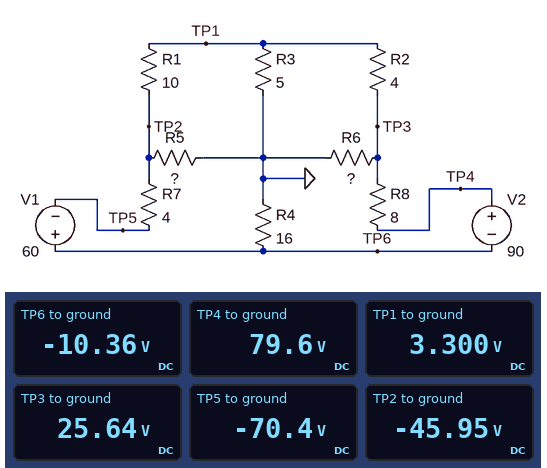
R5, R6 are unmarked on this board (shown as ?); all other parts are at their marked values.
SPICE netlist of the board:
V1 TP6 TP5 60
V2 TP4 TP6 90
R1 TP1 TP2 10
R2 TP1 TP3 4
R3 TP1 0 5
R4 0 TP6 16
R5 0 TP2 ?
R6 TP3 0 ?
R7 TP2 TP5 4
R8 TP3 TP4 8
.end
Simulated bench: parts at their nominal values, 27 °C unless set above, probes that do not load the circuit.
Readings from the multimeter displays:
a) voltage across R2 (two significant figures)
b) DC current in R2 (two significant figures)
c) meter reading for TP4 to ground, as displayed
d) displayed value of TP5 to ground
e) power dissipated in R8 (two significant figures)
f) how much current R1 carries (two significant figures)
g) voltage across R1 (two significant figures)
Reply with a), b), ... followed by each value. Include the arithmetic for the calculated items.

a) 25.64 V - 3.3 V = 22 V
b) (25.64 V - 3.3 V) / 4 Ω = 5.6 A
c) 79.6 V
d) -70.4 V
e) (79.6 V - 25.64 V)^2 / 8 Ω = 360 W
f) (3.3 V - (-45.95 V)) / 10 Ω = 4.9 A
g) 3.3 V - (-45.95 V) = 49 V
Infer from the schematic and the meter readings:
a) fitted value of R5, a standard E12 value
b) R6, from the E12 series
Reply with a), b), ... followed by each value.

a) 39 Ω
b) 22 Ω
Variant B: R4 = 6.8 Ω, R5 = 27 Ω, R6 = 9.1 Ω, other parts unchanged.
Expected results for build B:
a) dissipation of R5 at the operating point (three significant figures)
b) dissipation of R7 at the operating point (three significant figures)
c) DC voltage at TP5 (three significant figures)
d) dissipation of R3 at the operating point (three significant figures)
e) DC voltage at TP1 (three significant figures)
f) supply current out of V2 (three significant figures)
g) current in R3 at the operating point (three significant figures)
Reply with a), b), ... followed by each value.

a) 70.6 W
b) 153 W
c) -68.4 V
d) 899 mW
e) 2.12 V
f) 7.43 A
g) 424 mA
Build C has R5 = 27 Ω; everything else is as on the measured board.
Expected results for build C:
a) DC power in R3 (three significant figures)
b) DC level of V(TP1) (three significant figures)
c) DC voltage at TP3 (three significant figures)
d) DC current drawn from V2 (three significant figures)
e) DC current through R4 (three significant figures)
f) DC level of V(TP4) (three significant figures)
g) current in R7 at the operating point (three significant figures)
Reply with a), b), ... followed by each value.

a) 3.92 W
b) 4.43 V
c) 26.9 V
d) 6.85 A
e) 518 mA
f) 81.7 V
g) 6.33 A
